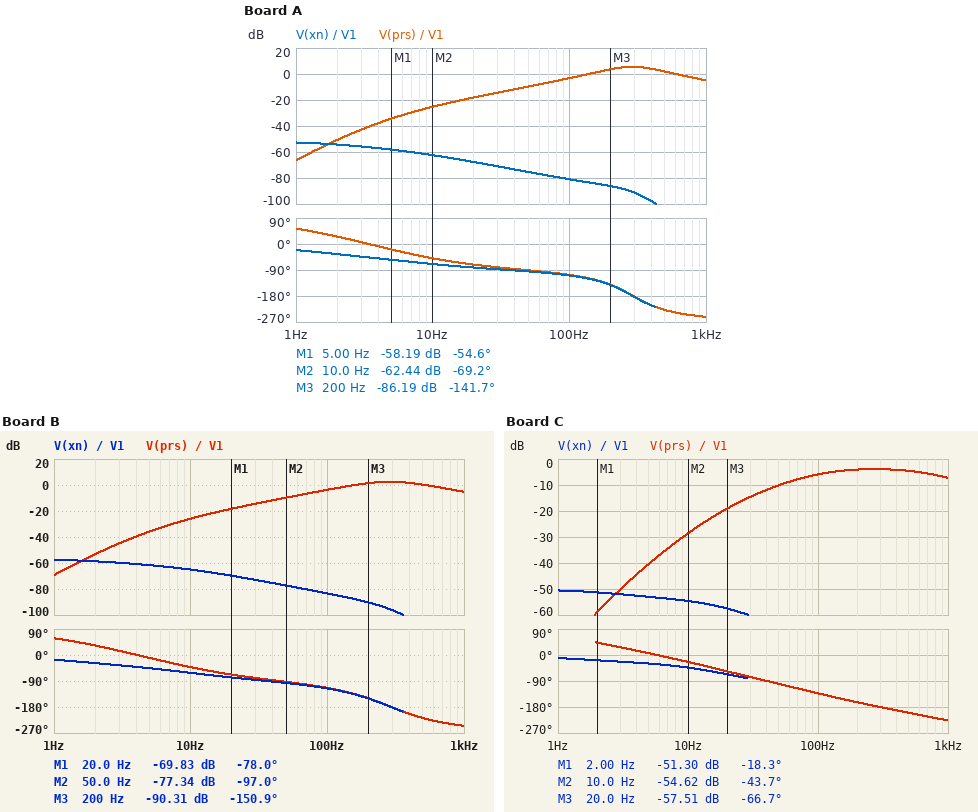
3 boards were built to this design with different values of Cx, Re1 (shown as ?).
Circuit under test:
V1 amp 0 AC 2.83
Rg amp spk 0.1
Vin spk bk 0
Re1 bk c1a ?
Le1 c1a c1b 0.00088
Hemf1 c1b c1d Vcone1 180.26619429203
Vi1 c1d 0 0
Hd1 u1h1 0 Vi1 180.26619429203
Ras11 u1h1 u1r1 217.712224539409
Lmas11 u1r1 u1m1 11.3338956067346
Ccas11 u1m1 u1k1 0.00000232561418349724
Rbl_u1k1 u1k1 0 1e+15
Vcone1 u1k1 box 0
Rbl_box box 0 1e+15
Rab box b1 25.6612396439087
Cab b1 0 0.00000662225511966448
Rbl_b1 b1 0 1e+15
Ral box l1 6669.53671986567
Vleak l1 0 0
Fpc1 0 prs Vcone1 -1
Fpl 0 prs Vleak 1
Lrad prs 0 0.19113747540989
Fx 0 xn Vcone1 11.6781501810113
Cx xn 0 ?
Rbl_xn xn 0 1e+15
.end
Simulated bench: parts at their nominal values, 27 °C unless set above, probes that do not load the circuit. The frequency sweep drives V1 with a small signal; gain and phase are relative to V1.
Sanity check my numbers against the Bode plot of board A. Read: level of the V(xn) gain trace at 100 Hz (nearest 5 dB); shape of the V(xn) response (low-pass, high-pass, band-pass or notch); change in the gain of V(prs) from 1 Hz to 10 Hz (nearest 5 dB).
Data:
-80 dB
low-pass
40 dB
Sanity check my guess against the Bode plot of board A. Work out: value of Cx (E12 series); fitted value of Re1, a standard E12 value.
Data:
1.2 F
1.5 Ω
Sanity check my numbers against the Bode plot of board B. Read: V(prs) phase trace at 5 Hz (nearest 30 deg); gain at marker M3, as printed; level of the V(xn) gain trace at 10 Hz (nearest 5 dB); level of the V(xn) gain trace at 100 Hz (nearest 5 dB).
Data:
0 deg
-90.31 dB
-65 dB
-85 dB
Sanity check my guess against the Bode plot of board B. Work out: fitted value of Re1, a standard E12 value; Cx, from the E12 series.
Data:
2.2 Ω
1.5 F
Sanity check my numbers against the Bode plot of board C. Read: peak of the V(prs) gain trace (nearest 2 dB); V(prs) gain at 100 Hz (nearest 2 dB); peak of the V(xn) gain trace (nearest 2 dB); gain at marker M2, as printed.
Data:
-4 dB
-6 dB
-50 dB
-54.62 dB
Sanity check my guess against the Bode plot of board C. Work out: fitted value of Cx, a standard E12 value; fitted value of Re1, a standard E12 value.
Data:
330 mF
4.7 Ω
